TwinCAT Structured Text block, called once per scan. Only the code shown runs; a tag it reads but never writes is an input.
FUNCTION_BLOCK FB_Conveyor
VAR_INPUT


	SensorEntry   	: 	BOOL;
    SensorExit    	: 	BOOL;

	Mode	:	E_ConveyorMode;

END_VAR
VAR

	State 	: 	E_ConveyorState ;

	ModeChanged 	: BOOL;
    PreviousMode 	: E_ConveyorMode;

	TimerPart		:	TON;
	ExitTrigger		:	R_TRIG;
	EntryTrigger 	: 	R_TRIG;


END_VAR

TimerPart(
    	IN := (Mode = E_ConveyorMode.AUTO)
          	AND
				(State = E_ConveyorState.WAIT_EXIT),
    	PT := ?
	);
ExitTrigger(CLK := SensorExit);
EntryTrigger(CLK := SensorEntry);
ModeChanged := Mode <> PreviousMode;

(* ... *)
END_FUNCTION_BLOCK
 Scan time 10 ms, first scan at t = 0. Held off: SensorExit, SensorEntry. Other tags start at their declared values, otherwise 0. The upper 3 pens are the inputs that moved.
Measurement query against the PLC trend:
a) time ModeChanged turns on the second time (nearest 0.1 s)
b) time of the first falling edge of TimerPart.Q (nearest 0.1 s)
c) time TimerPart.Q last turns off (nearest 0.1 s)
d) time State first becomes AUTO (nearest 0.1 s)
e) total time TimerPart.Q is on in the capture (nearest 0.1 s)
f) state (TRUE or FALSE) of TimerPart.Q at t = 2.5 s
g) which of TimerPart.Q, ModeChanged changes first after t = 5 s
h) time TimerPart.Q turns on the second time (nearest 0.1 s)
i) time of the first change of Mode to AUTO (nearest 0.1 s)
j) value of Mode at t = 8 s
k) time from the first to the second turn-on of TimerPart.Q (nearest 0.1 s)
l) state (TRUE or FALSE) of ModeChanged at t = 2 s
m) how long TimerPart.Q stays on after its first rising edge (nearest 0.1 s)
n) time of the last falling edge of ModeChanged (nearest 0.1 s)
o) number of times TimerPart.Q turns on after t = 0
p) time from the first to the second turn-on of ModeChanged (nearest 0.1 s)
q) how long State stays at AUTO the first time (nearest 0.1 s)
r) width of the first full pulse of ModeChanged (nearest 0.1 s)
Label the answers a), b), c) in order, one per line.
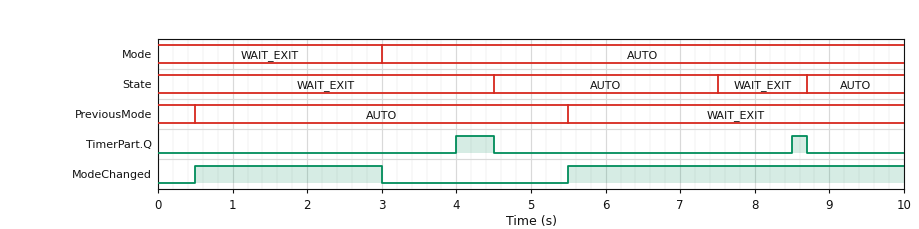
a) 5.5 s
b) 4.5 s
c) 8.7 s
d) 4.5 s
e) 0.7 s
f) FALSE
g) ModeChanged
h) 8.5 s
i) 3.0 s
j) AUTO
k) 4.5 s
l) TRUE
m) 0.5 s
n) 3.0 s
o) 2
p) 5.0 s
q) 3.0 s
r) 2.5 s
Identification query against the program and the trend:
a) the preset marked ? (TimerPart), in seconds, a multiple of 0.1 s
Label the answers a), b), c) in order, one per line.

a) 1.0 s
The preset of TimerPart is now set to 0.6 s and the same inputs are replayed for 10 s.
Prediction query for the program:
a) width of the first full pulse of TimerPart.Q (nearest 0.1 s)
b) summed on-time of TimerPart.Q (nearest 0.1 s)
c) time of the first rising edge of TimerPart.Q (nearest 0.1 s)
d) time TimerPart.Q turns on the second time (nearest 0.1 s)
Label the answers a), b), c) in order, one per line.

a) 0.9 s
b) 1.5 s
c) 3.6 s
d) 8.1 s
